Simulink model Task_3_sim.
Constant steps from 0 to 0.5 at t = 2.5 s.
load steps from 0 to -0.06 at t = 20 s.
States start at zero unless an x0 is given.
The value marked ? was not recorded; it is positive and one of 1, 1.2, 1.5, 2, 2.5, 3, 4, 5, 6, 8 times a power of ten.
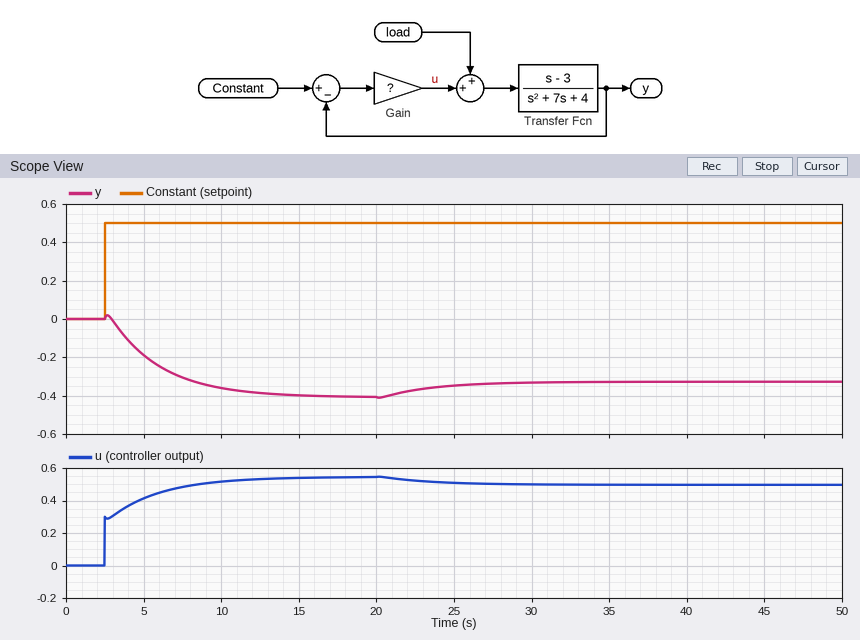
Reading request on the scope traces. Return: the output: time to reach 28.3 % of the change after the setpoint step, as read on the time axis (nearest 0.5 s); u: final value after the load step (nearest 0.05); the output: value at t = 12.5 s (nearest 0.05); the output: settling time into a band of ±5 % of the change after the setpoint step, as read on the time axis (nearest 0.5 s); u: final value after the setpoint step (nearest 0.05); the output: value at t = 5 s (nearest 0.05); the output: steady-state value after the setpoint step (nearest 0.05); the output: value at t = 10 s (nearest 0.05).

4.0 s
0.50
-0.40
13.0 s
0.55
-0.20
-0.40
-0.35
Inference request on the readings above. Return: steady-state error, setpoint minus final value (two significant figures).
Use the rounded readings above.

0.90
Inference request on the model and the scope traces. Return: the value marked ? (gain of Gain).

0.6
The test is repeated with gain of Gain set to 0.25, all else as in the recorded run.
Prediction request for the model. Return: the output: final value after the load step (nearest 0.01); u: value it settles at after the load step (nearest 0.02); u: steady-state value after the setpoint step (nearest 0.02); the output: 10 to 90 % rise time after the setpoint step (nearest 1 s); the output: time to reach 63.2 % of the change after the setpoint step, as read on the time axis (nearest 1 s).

-0.06
0.14
0.16
5 s
5 s
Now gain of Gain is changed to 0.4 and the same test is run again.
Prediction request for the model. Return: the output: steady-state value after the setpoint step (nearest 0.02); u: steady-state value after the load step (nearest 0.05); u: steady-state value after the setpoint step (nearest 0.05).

-0.22
0.25
0.30
